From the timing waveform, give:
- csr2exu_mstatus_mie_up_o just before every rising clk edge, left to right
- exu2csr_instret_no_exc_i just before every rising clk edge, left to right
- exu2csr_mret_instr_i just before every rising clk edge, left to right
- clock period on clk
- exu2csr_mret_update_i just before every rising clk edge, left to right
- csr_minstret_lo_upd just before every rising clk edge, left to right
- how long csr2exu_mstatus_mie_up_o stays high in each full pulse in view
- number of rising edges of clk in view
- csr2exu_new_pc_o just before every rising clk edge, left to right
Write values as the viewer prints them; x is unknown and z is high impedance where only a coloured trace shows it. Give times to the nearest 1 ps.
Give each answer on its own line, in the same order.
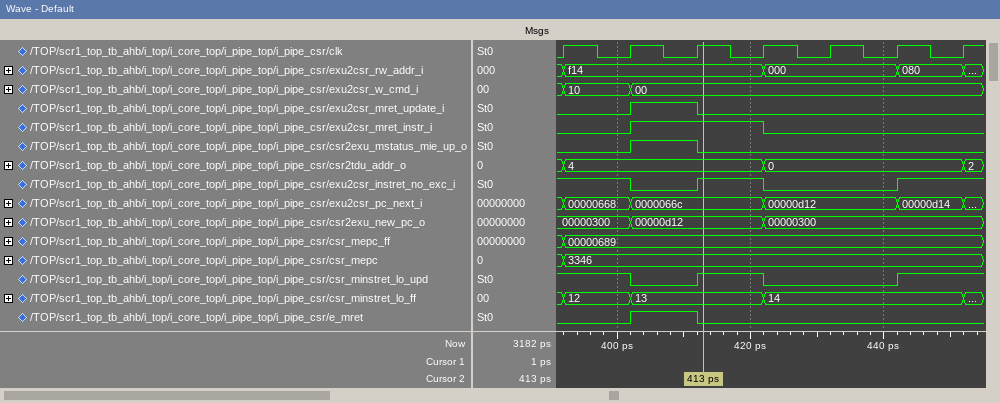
0 0 1 0 0 0 0
1 1 0 1 0 0 1
0 0 1 1 0 0 0
10 ps
0 0 1 0 0 0 0
1 1 0 1 0 0 1
10 ps
7
00000300, 00000300, 00000d12, 00000d12, 00000300, 00000300, 00000300
